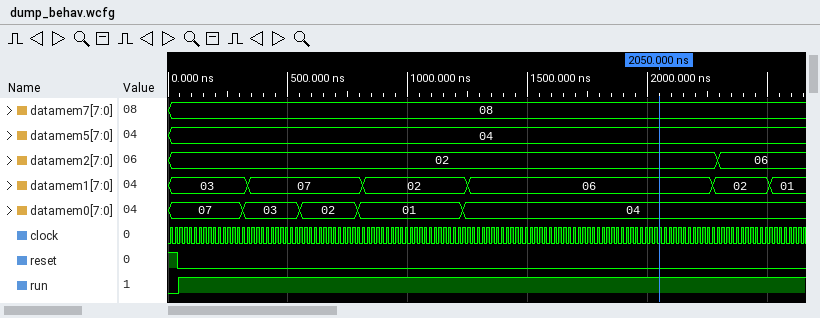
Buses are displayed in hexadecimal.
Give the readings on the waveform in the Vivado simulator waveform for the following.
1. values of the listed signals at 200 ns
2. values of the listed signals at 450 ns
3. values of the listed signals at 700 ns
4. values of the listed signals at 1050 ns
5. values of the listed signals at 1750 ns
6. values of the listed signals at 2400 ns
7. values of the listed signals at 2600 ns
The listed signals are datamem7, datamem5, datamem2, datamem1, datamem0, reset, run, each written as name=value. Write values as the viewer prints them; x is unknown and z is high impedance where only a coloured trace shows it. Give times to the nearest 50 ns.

datamem7=08, datamem5=04, datamem2=02, datamem1=03, datamem0=07, reset=0, run=1
datamem7=08, datamem5=04, datamem2=02, datamem1=07, datamem0=03, reset=0, run=1
datamem7=08, datamem5=04, datamem2=02, datamem1=07, datamem0=02, reset=0, run=1
datamem7=08, datamem5=04, datamem2=02, datamem1=02, datamem0=01, reset=0, run=1
datamem7=08, datamem5=04, datamem2=02, datamem1=06, datamem0=04, reset=0, run=1
datamem7=08, datamem5=04, datamem2=06, datamem1=02, datamem0=04, reset=0, run=1
datamem7=08, datamem5=04, datamem2=06, datamem1=01, datamem0=04, reset=0, run=1
